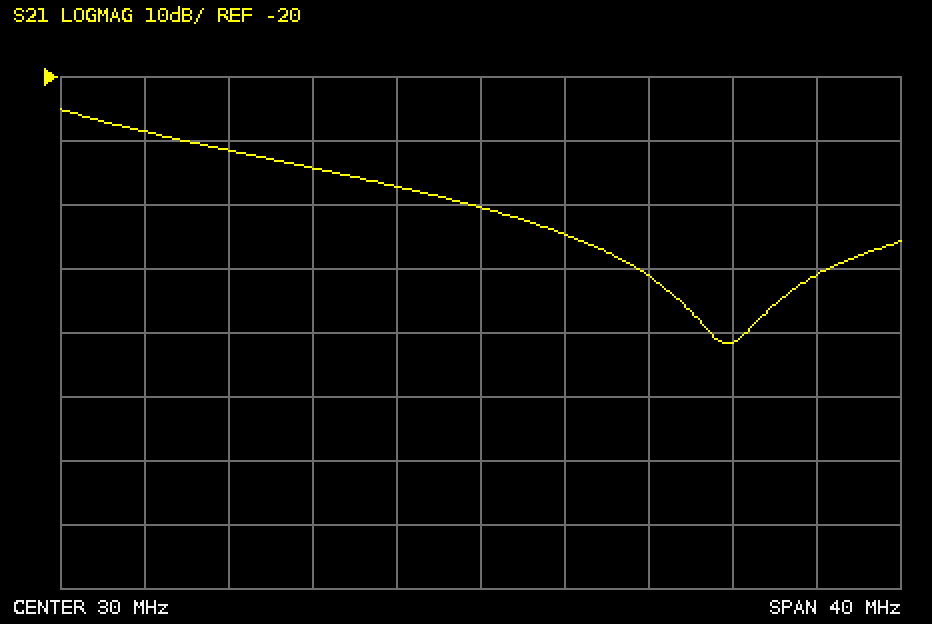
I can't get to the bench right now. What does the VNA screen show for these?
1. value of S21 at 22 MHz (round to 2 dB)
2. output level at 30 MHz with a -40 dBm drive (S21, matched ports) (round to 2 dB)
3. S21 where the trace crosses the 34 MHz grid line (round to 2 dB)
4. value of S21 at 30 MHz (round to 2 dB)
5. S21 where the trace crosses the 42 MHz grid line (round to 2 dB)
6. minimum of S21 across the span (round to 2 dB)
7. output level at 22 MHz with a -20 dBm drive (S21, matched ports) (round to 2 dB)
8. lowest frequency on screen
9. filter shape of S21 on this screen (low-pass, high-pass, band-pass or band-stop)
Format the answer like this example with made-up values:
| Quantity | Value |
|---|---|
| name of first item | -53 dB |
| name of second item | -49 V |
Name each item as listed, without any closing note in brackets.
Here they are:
| Quantity | Value |
|---|---|
| value of S21 at 22 MHz | -34 dB |
| output level at 30 MHz with a -40 dBm drive (S21, matched ports) | -80 dBm |
| S21 where the trace crosses the 34 MHz grid line | -44 dB |
| value of S21 at 30 MHz | -40 dB |
| S21 where the trace crosses the 42 MHz grid line | -62 dB |
| minimum of S21 across the span | -62 dB |
| output level at 22 MHz with a -20 dBm drive (S21, matched ports) | -54 dBm |
| lowest frequency on screen | 10 MHz |
| filter shape of S21 on this screen | low-pass |
